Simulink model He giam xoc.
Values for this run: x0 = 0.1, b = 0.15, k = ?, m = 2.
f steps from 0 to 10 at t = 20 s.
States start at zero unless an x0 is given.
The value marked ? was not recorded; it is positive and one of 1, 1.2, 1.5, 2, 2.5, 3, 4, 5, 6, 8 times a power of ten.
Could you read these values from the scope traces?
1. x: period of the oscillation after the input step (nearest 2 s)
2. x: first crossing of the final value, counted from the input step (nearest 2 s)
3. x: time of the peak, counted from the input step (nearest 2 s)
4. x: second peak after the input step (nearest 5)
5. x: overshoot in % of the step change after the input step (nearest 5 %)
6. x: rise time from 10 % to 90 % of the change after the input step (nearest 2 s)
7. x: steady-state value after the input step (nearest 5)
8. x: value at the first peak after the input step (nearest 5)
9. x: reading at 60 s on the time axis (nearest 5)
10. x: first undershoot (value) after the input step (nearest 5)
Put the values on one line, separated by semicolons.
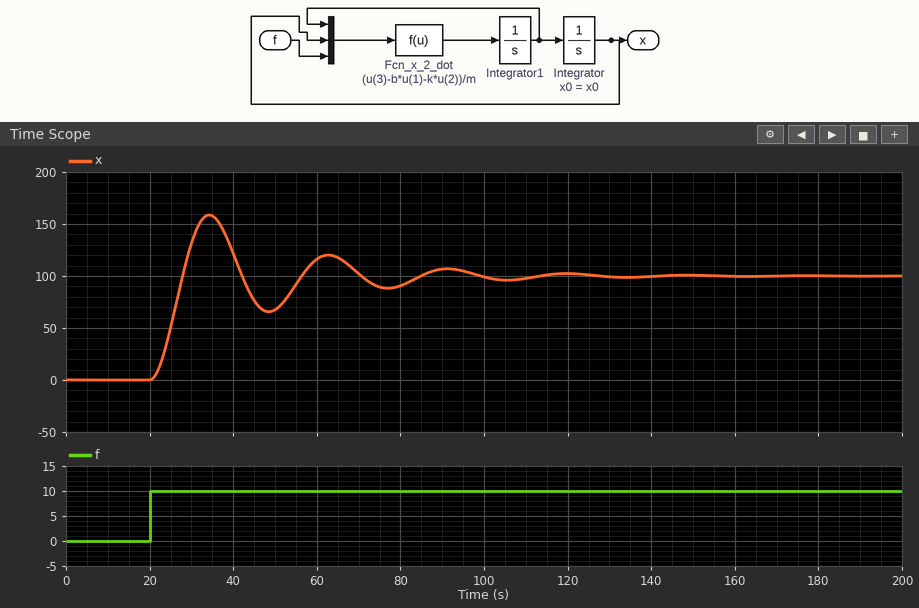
28 s; 8 s; 14 s; 120; 60 %; 6 s; 100; 160; 115; 65
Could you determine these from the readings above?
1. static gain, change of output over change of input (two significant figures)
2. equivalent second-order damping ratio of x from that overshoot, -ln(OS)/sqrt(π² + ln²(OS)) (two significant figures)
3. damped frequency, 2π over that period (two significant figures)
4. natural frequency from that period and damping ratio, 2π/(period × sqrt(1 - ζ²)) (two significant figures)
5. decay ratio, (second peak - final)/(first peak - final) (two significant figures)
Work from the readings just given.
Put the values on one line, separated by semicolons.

10; 0.16; 0.22 rad/s; 0.23 rad/s; 0.33
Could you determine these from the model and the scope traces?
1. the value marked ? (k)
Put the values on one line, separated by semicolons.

0.1
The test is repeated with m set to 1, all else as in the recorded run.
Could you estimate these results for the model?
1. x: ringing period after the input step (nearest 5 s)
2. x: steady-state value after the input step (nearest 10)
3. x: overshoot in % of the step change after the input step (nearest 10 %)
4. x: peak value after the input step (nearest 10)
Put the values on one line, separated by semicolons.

20 s; 100; 50 %; 150
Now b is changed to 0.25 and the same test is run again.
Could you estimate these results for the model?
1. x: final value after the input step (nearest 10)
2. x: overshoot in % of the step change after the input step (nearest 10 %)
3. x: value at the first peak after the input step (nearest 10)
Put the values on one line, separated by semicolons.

100; 40 %; 140
